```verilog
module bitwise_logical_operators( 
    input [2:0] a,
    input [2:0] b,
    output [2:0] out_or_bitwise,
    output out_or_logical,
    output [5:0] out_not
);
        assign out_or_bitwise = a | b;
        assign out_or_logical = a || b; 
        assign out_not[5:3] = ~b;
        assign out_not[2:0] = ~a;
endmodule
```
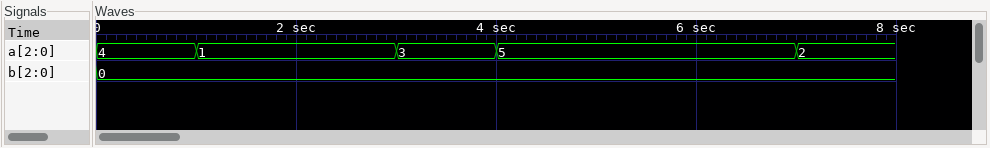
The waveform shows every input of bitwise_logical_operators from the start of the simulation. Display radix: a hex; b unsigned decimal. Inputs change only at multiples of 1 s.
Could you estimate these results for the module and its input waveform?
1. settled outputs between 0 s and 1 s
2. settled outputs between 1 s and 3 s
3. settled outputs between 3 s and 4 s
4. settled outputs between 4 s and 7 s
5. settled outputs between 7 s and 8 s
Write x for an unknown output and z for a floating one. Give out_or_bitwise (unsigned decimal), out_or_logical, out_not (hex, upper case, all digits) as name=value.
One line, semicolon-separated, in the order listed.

out_or_bitwise=4, out_or_logical=1, out_not=3B; out_or_bitwise=1, out_or_logical=1, out_not=3E; out_or_bitwise=3, out_or_logical=1, out_not=3C; out_or_bitwise=5, out_or_logical=1, out_not=3A; out_or_bitwise=2, out_or_logical=1, out_not=3D
